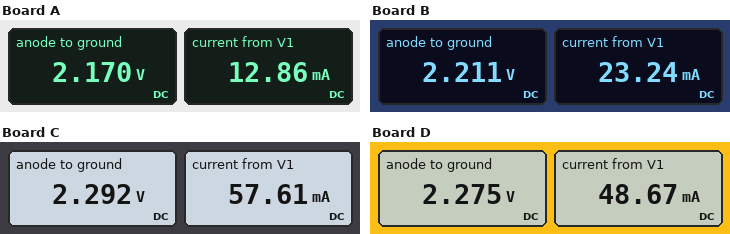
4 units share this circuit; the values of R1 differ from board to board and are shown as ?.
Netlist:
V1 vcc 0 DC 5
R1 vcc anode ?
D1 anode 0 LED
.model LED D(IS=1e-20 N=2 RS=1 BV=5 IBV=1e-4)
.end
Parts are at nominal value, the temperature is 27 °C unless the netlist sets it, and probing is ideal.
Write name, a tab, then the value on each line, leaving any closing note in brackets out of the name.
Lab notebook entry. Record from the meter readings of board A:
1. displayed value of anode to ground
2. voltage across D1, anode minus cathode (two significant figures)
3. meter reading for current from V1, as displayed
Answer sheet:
displayed value of anode to ground	2.170 V
voltage across D1, anode minus cathode	2.2 V
meter reading for current from V1, as displayed	12.86 mA
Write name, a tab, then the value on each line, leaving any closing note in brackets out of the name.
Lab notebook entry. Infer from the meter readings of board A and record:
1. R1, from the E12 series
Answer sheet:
R1, from the E12 series	220 Ω
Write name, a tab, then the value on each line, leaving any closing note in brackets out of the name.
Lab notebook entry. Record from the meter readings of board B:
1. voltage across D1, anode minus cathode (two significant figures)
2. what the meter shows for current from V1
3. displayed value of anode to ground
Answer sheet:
voltage across D1, anode minus cathode	2.2 V
what the meter shows for current from V1	23.24 mA
displayed value of anode to ground	2.211 V
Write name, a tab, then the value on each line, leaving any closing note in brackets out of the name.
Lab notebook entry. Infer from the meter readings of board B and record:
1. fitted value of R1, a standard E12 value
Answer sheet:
fitted value of R1, a standard E12 value	120 Ω
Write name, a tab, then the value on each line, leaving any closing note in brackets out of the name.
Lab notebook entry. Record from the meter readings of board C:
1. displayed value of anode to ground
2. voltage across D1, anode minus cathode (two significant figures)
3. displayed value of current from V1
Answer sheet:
displayed value of anode to ground	2.292 V
voltage across D1, anode minus cathode	2.3 V
displayed value of current from V1	57.61 mA
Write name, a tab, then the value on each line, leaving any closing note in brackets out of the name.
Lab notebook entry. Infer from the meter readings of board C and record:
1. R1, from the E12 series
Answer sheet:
R1, from the E12 series	47 Ω
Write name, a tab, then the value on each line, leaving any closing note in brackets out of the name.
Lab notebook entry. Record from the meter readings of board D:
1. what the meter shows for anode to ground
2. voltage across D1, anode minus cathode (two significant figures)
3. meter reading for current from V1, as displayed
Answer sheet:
what the meter shows for anode to ground	2.275 V
voltage across D1, anode minus cathode	2.3 V
meter reading for current from V1, as displayed	48.67 mA
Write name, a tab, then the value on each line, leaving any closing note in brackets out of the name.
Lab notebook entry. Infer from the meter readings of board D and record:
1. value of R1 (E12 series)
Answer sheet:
value of R1	56 Ω
